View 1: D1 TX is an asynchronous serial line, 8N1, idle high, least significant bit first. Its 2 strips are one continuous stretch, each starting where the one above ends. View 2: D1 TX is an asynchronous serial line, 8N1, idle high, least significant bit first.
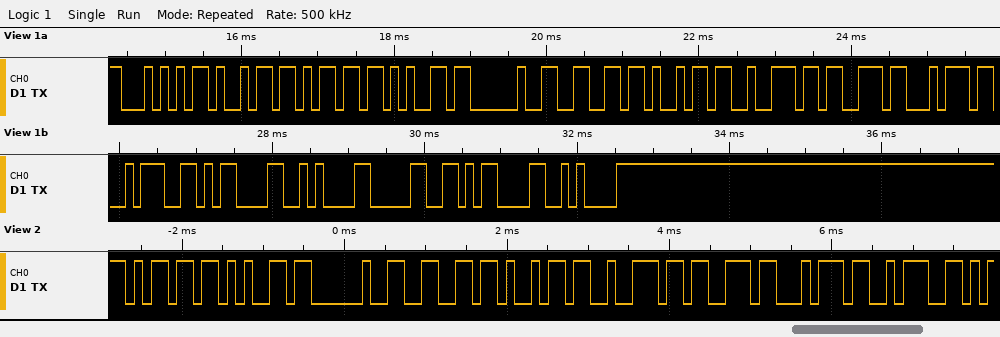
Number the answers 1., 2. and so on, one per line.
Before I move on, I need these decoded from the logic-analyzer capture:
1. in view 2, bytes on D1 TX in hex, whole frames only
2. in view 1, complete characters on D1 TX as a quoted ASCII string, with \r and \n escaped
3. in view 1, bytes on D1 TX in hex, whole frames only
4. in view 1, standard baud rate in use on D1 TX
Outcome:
1. 6D 65 20 66 69 72 73 74 3A
2. "Time first:\r\n0\r\n"
3. 54 69 6D 65 20 66 69 72 73 74 3A 0D 0A 30 0D 0A
4. 9600 baud
